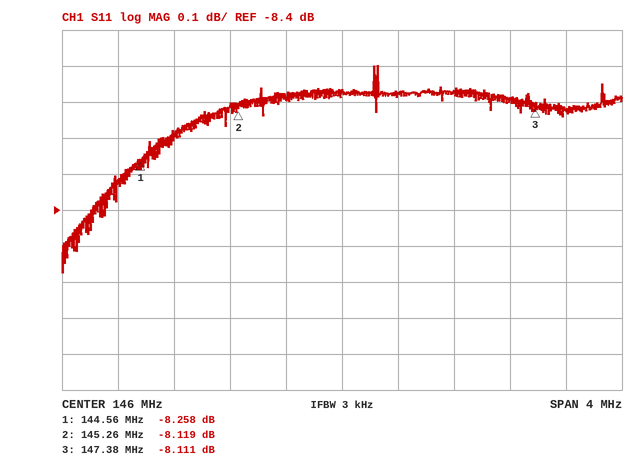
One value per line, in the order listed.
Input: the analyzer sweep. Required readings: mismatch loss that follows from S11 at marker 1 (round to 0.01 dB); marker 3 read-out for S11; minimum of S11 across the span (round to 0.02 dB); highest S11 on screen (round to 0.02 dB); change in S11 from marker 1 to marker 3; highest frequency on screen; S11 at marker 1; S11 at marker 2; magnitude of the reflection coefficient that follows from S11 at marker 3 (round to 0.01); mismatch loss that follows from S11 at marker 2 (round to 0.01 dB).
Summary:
0.70 dB
-8.111 dB
-8.58 dB
-8.00 dB
0.147 dB
148 MHz
-8.258 dB
-8.119 dB
0.39
0.73 dB
